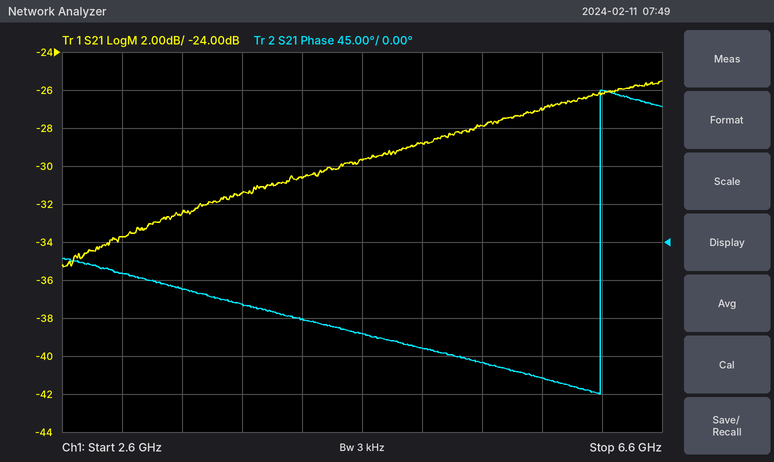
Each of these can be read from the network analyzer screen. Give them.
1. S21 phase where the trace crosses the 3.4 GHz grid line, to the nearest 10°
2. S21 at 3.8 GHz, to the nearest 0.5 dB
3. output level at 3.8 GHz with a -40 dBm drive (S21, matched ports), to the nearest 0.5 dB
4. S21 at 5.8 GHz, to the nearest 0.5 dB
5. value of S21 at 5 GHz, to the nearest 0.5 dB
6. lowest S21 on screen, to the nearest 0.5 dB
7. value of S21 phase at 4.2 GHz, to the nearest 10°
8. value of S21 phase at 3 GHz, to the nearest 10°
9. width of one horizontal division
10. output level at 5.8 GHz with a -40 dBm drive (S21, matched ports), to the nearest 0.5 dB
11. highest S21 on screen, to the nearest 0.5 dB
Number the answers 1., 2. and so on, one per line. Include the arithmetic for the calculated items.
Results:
1. -60°
2. -31.5 dB
3. -40 dBm + (-31.5 dB) = -71.5 dBm
4. -27.0 dB
5. -29.0 dB
6. -35.5 dB
7. -90°
8. -40°
9. 400 MHz
10. -40 dBm + (-27.0 dB) = -67.0 dBm
11. -25.5 dB
